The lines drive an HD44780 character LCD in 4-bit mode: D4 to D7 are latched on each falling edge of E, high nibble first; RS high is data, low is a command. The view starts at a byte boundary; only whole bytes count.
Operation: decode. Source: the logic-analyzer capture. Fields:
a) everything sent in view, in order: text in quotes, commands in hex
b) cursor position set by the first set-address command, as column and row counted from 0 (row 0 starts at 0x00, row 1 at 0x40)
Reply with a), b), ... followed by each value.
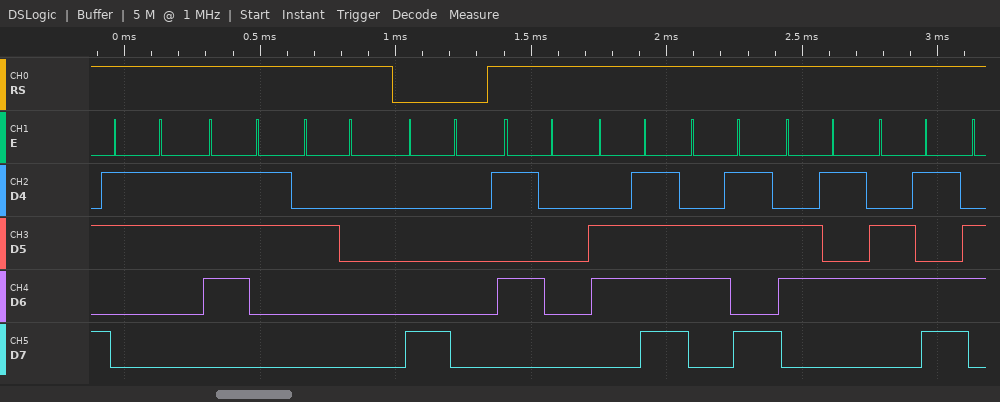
a) "3s " 0x80 "Pokem"
b) column 0, row 0
